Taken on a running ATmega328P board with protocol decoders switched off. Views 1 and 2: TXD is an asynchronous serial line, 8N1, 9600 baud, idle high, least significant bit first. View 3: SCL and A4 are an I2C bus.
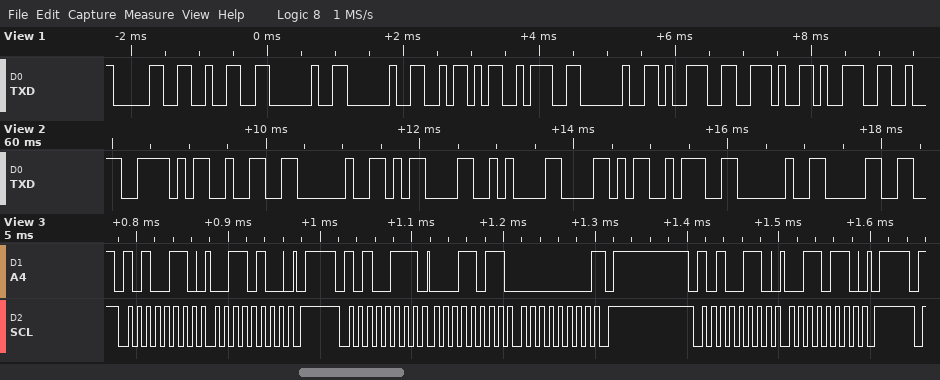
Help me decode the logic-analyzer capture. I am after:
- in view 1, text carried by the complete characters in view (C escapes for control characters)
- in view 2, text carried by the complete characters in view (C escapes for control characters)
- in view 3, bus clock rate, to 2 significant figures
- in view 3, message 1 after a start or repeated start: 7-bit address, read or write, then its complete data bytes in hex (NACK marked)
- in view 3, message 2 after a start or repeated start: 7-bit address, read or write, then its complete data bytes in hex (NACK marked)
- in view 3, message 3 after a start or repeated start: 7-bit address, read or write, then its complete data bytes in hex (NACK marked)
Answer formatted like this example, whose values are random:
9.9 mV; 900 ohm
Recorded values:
"02  Z: 9.9"; "^2 \r\nX: 0"; 100 kHz; 0x53 write: 34; 0x53 read: 1B 00 NACK; 0x53 write: 36
